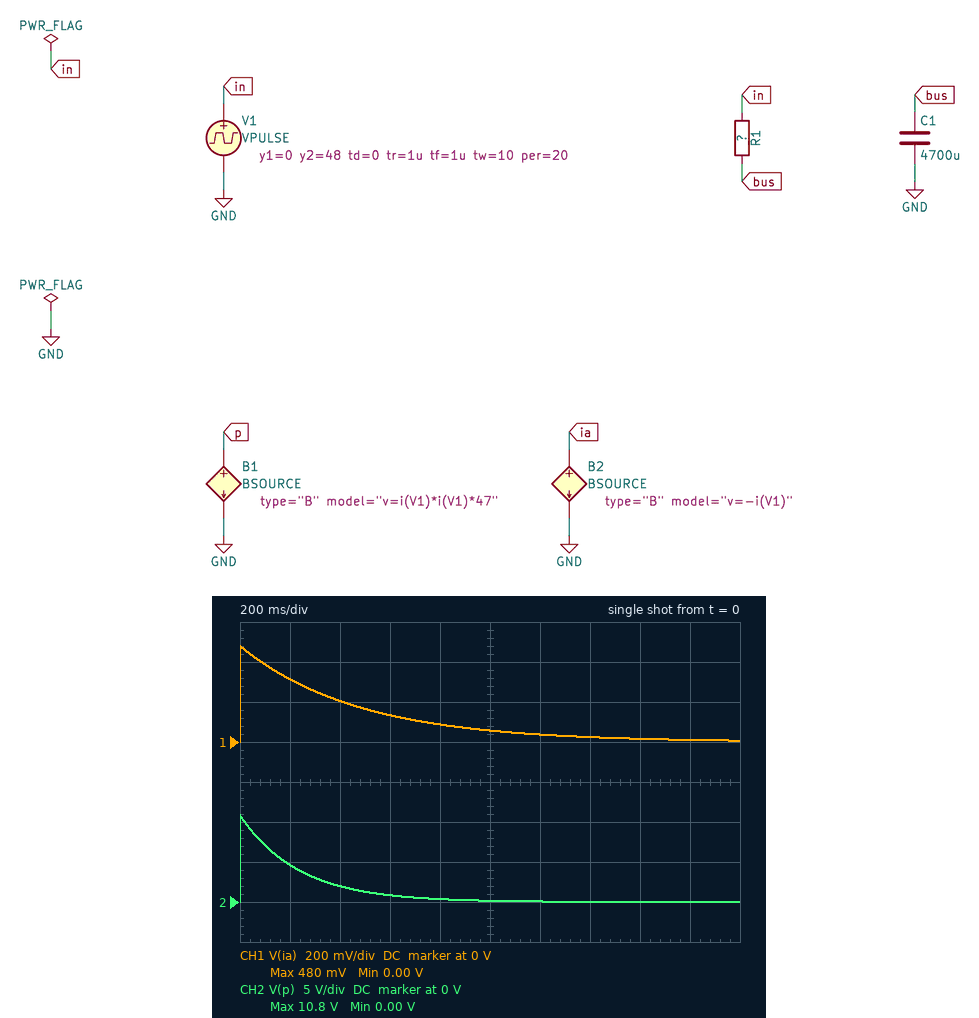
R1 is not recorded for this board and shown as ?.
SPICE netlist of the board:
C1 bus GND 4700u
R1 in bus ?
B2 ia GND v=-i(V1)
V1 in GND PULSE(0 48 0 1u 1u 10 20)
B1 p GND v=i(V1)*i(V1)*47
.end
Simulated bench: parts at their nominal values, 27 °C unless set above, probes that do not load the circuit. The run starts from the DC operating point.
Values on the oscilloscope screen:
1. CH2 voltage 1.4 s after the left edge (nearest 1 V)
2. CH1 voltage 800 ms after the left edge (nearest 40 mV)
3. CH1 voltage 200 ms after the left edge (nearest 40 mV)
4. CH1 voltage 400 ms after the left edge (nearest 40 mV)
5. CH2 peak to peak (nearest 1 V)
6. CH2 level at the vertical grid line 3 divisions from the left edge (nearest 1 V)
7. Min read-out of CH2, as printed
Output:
0 V
80 mV
320 mV
200 mV
11 V
1 V
0.00 V
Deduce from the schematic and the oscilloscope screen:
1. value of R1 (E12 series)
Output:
100 Ω
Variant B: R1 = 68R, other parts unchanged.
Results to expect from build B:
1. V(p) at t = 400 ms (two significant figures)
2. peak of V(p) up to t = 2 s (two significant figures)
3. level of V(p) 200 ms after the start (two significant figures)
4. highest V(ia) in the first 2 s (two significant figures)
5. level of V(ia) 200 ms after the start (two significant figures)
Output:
1.9 V
23 V
6.7 V
710 mV
380 mV
